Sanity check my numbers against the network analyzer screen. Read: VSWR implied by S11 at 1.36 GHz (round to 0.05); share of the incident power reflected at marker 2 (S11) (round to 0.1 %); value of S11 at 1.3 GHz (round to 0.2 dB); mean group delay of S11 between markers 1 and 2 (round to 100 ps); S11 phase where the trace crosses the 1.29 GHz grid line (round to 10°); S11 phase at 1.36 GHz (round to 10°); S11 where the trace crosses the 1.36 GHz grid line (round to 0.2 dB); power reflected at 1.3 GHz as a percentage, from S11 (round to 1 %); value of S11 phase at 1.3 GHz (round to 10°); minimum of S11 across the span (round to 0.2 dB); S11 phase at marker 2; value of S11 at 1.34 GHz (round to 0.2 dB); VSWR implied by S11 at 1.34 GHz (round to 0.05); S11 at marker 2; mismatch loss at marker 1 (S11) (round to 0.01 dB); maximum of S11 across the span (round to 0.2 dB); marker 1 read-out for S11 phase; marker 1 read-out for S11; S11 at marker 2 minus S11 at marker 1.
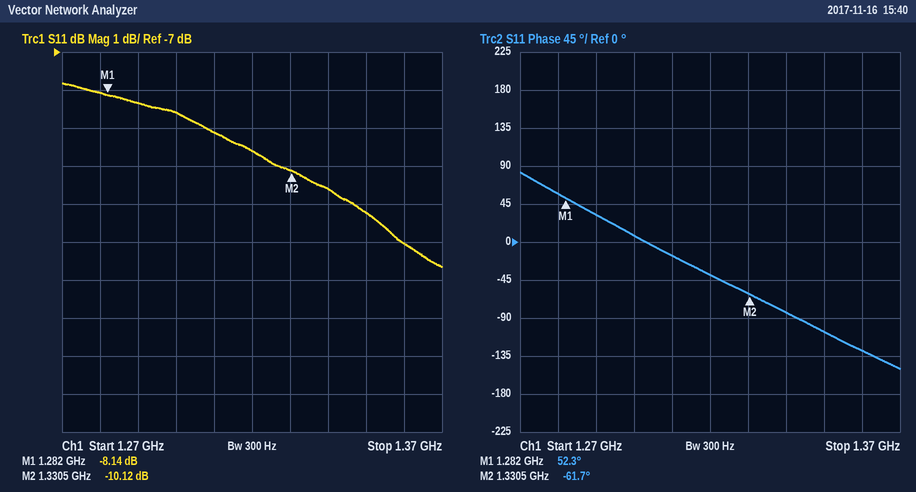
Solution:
1.65
9.7 %
-8.6 dB
6.5 ns
30°
-130°
-12.0 dB
14 %
10°
-12.6 dB
-61.7°
-10.6 dB
1.85
-10.12 dB
0.72 dB
-7.8 dB
52.3°
-8.14 dB
-1.98 dB
